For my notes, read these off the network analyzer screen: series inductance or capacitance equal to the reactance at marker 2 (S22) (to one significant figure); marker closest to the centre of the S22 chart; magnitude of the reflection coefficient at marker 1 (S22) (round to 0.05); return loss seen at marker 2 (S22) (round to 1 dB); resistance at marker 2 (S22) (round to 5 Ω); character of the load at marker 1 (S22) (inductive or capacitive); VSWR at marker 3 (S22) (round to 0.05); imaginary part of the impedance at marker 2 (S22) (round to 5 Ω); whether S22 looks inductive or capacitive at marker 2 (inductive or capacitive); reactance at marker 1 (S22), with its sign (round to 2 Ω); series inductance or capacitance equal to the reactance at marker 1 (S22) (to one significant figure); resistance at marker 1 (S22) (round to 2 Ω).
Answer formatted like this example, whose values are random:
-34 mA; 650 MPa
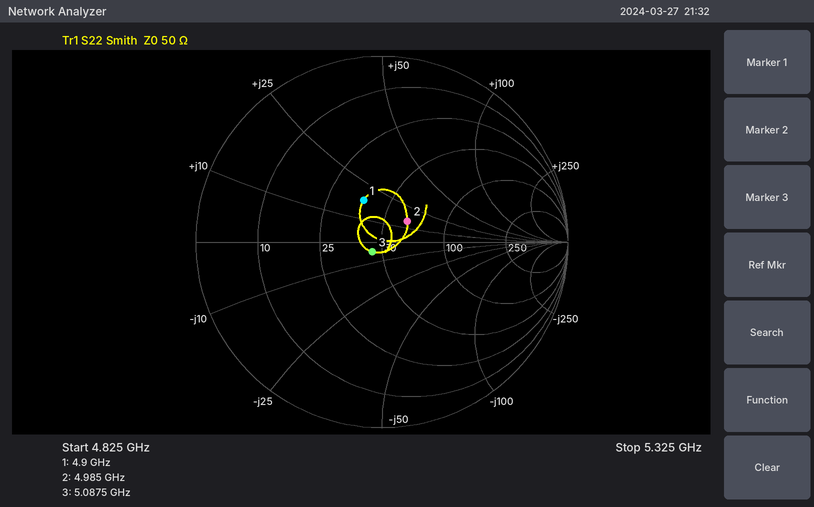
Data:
500 pH; marker 3; 0.25; 15 dB; 65 Ω; inductive; 1.15; +15 Ω; inductive; +18 Ω; 600 pH; 38 Ω
